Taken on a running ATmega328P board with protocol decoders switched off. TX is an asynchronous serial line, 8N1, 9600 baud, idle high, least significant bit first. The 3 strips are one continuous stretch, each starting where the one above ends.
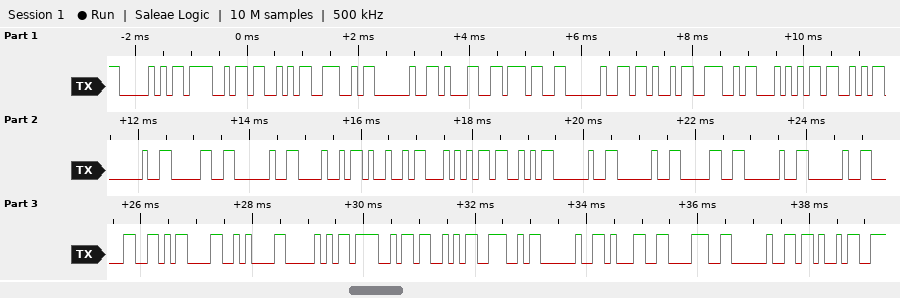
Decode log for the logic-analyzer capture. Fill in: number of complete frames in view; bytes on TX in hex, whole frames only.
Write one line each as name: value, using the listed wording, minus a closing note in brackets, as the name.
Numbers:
number of complete frames in view: 36
bytes on TX in hex, whole frames only: 50 4F 53 4E 20 31 37 20 4B 4E 54 53 20 30 20 48 49 54 53 20 20 30 20 20 30 0D 0A 50 4F 53 4E 20 31 38 20 4B
